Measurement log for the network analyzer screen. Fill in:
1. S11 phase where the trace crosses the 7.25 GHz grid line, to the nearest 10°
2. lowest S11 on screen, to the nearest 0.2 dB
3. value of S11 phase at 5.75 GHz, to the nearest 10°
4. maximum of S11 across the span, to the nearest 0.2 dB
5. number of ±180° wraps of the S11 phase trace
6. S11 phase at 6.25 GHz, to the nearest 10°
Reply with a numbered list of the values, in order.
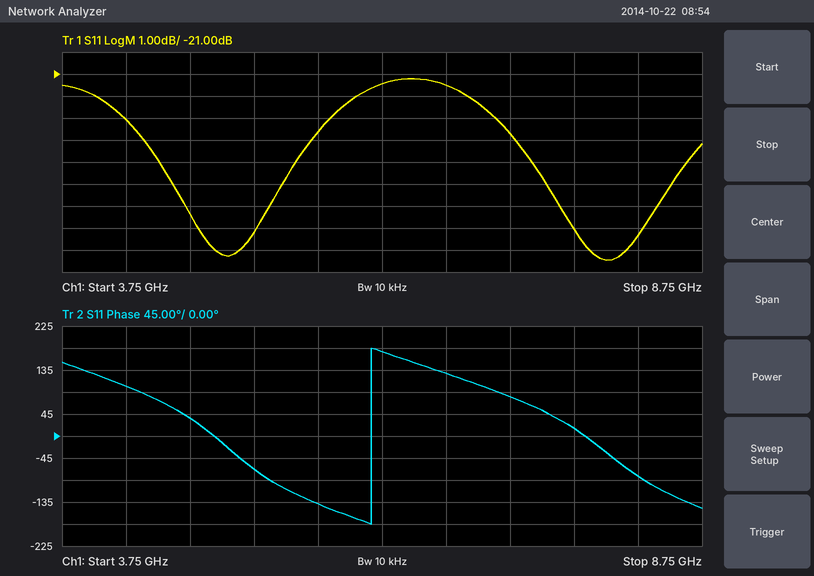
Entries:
1. 80°
2. -29.4 dB
3. -140°
4. -21.2 dB
5. 1
6. 170°
